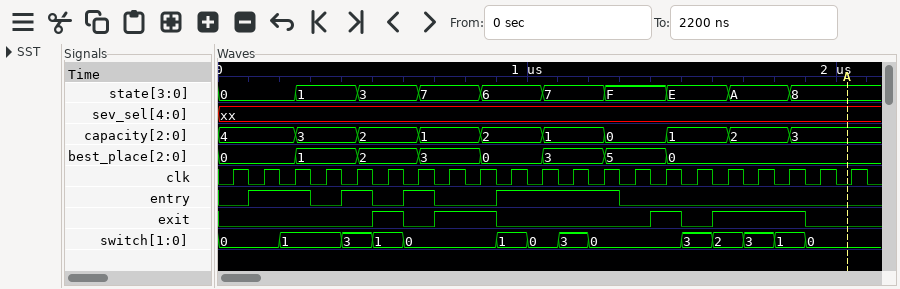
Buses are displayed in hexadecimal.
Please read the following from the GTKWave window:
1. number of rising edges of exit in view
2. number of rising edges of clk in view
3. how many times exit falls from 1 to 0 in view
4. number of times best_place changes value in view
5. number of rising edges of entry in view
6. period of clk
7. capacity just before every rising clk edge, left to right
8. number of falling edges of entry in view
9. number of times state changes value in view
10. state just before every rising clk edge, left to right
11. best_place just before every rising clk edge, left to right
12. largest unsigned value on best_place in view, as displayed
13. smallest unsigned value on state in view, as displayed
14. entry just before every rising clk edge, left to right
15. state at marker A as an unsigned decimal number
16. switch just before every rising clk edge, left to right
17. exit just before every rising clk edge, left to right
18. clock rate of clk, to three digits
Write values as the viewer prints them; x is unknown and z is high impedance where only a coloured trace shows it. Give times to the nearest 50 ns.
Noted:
4
21
4
7
4
100 ns
4, 4, 4, 3, 3, 2, 2, 1, 1, 2, 2, 1, 1, 0, 0, 1, 1, 2, 2, 3, 3
4
9
0, 0, 0, 1, 1, 3, 3, 7, 7, 6, 6, 7, 7, F, F, E, E, A, A, 8, 8
0, 0, 0, 1, 1, 2, 2, 3, 3, 0, 0, 3, 3, 5, 5, 0, 0, 0, 0, 0, 0
5
0
0 1 1 0 1 0 1 0 0 1 1 1 1 0 0 0 0 0 0 0 0
8
0, 0, 1, 1, 3, 1, 0, 0, 0, 1, 0, 3, 0, 0, 0, 3, 2, 3, 1, 0, 0
0 0 0 0 0 1 0 1 1 0 0 0 0 0 1 0 1 1 1 0 0
10.0 MHz
